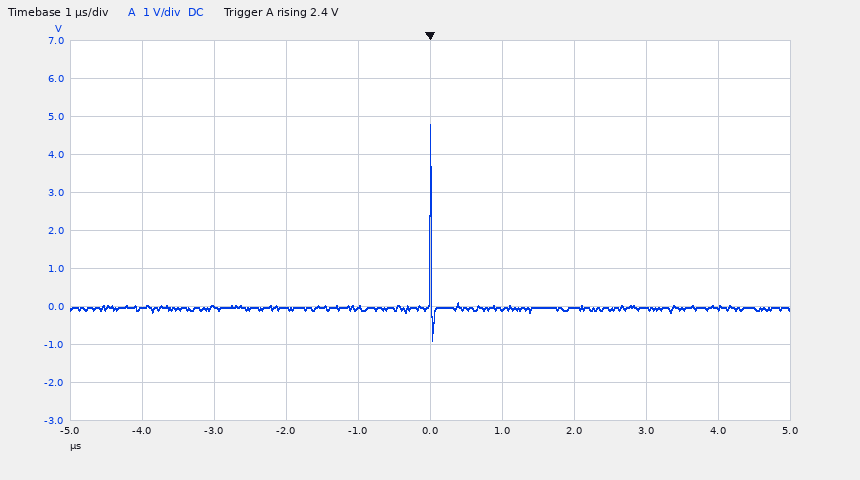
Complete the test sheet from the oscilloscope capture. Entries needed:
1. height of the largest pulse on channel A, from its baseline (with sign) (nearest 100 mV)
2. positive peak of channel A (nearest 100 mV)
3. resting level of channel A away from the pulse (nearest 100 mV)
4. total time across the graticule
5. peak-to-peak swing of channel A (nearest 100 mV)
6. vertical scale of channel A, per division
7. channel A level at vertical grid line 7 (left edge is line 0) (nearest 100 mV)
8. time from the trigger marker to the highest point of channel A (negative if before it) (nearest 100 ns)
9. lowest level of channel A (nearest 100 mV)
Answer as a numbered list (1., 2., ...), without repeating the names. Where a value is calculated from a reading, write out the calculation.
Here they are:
1. 4.8 V − (0.0 V) = +4.8 V
2. 4.8 V
3. 0.0 V
4. 10 µs
5. 4.8 V − (-900 mV) = 5.7 V
6. 1 V
7. 0.0 V
8. 0.0 µs
9. -900 mV
